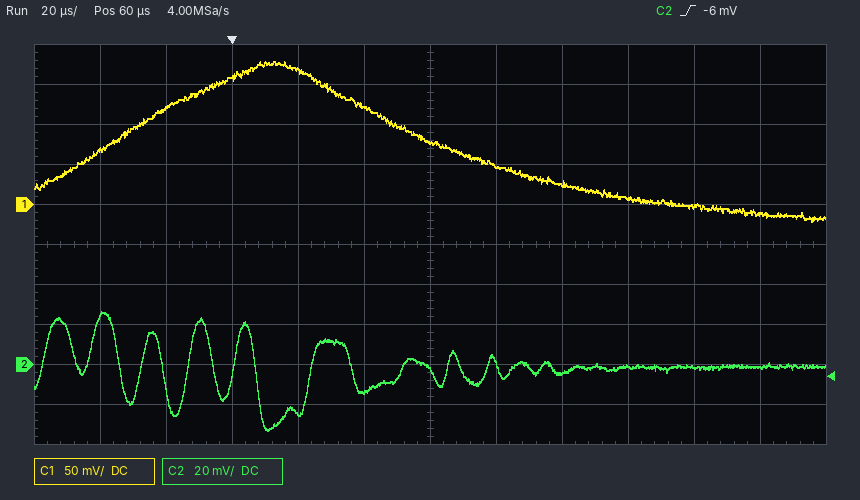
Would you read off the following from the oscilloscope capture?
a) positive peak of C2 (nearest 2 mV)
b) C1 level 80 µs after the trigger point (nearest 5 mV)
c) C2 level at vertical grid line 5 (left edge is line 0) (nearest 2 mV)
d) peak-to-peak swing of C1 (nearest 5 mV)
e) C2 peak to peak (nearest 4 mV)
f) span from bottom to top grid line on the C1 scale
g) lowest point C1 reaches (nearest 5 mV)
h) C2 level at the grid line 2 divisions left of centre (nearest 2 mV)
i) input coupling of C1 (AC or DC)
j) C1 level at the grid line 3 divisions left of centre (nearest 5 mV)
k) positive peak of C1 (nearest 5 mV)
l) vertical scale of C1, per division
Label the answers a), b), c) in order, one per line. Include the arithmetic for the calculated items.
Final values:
a) 26 mV
b) 50 mV
c) -14 mV
d) 180 mV − (-20 mV) = 200 mV
e) 60 mV
f) 500 mV
g) -20 mV
h) -24 mV
i) DC
j) 160 mV
k) 180 mV
l) 50 mV
